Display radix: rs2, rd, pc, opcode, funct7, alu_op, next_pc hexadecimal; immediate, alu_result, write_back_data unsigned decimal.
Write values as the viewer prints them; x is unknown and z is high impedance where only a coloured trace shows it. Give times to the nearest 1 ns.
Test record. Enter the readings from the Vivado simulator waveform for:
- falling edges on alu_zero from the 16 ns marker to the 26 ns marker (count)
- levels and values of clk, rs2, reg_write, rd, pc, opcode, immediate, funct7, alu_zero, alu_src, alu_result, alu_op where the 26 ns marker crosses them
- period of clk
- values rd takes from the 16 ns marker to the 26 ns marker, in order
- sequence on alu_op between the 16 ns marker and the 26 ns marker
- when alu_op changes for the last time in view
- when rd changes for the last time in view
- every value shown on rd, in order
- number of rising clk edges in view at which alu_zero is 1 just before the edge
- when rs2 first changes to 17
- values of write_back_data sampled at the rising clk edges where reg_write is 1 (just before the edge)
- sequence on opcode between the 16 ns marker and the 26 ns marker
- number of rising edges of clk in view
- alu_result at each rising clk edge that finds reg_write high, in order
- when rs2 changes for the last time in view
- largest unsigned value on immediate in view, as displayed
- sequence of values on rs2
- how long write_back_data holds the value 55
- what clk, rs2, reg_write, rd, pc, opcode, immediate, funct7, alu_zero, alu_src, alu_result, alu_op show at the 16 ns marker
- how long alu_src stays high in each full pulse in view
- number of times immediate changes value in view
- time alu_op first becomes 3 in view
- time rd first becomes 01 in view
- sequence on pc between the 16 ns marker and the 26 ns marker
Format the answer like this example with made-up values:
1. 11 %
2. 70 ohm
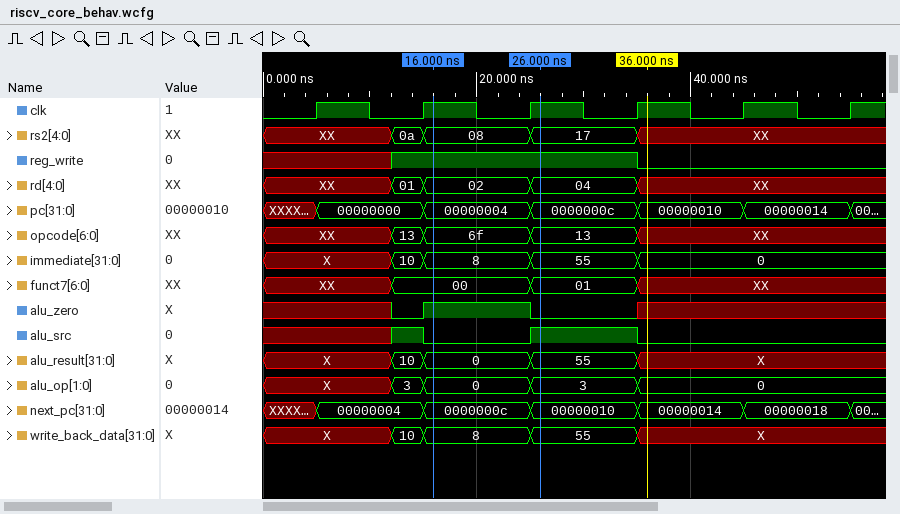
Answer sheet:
1. 1
2. clk=1, rs2=17, reg_write=1, rd=04, pc=0000000c, opcode=13, immediate=55, funct7=01, alu_zero=0, alu_src=1, alu_result=55, alu_op=3
3. 10 ns
4. 02, 04
5. 0, 3
6. 35 ns
7. 35 ns
8. XX, 01, 02, 04, XX
9. 1
10. 25 ns
11. 10, 8, 55
12. 6f, 13
13. 6
14. 10, 0, 55
15. 35 ns
16. 55
17. XX, 0a, 08, 17, XX
18. 10 ns
19. clk=1, rs2=08, reg_write=1, rd=02, pc=00000004, opcode=6f, immediate=8, funct7=00, alu_zero=1, alu_src=0, alu_result=0, alu_op=0
20. 10 ns
21. 4
22. 12 ns
23. 12 ns
24. 00000004, 0000000c
